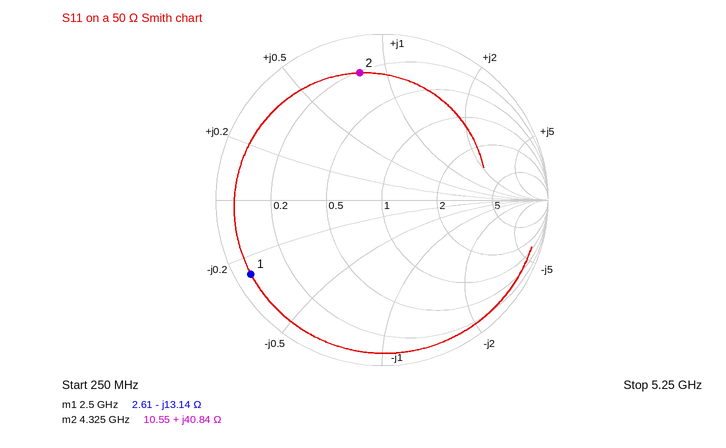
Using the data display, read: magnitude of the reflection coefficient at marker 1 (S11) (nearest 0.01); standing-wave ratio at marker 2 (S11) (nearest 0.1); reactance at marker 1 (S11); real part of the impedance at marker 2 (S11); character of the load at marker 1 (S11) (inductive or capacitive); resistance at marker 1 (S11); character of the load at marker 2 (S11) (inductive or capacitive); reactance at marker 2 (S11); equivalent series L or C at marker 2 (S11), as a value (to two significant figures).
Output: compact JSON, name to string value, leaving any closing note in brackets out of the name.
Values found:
{"magnitude of the reflection coefficient at marker 1 (S11)": "0.91", "standing-wave ratio at marker 2 (S11)": "8.0", "reactance at marker 1": "-13.14 Ω", "real part of the impedance at marker 2": "10.55 Ω", "character of the load at marker 1 (S11)": "capacitive", "resistance at marker 1": "2.61 Ω", "character of the load at marker 2 (S11)": "inductive", "reactance at marker 2": "+40.84 Ω", "equivalent series L or C at marker 2 (S11), as a value": "1.5 nH"}
